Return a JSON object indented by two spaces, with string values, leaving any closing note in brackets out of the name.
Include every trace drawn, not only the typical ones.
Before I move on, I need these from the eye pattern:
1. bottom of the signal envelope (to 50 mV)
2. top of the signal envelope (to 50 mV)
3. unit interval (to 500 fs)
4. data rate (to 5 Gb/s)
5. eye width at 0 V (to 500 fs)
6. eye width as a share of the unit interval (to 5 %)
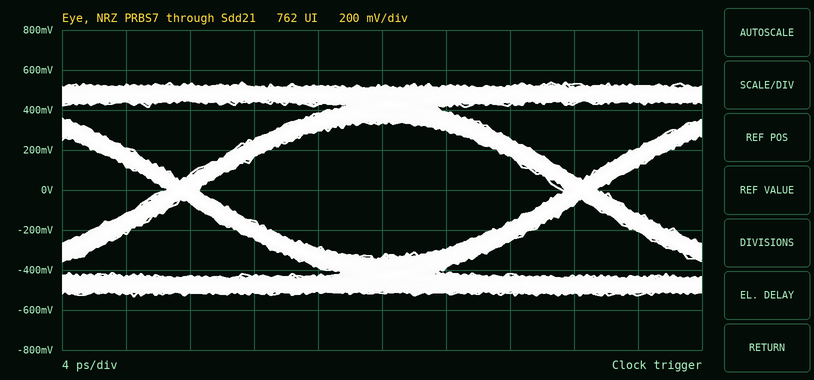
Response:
{
  "bottom of the signal envelope": "-550 mV",
  "top of the signal envelope": "550 mV",
  "unit interval": "25.0 ps",
  "data rate": "40 Gb/s",
  "eye width at 0 V": "22.5 ps",
  "eye width as a share of the unit interval": "90 %"
}
